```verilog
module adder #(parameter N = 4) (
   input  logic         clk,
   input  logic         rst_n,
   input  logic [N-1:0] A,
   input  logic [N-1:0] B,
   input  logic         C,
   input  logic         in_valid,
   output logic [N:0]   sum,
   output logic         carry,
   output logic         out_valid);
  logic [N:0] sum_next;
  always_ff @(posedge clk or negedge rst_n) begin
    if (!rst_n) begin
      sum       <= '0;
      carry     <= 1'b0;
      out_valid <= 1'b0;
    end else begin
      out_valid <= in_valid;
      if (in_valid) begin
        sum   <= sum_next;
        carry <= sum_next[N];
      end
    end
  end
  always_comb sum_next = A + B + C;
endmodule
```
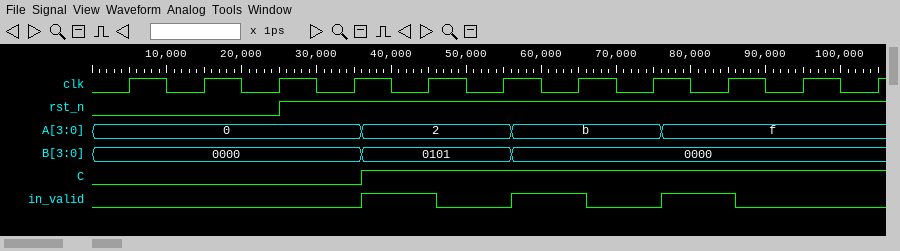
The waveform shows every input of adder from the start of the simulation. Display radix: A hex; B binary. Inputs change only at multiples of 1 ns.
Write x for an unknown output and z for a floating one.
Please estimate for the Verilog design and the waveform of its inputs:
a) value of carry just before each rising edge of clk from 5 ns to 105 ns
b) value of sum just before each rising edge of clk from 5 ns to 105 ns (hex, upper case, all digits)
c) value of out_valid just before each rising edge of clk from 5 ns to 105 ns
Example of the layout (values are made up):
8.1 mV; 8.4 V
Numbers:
0 0 0 0 0 0 0 0 0 1 1; 00, 00, 00, 00, 00, 08, 08, 0C, 0C, 10, 10; 0 0 0 0 0 1 0 1 0 1 0
